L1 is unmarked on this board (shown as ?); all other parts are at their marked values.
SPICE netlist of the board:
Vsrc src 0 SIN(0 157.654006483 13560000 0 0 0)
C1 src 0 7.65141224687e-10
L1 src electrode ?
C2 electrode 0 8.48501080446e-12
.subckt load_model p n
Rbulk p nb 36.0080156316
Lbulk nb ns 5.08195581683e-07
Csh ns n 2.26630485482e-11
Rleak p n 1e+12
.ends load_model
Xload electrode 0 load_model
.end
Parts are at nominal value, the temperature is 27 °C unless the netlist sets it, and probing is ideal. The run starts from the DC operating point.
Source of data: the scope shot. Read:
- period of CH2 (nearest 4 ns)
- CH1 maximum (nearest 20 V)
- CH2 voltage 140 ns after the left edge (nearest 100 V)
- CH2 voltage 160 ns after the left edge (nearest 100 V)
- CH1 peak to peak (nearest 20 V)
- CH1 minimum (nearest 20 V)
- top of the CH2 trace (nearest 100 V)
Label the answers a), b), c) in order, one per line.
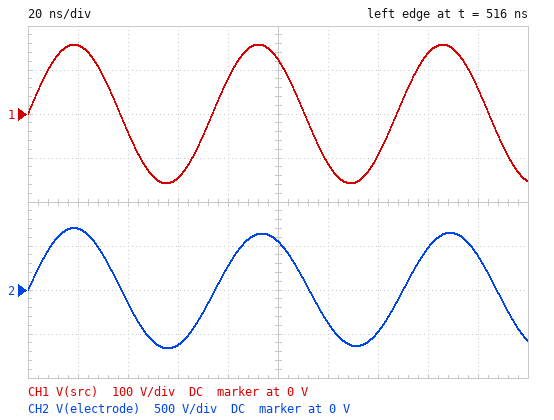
a) 76 ns
b) 160 V
c) -500 V
d) 500 V
e) 320 V
f) -160 V
g) 700 V
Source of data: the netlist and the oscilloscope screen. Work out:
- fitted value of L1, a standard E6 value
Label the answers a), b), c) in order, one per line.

a) 3.3 µH
